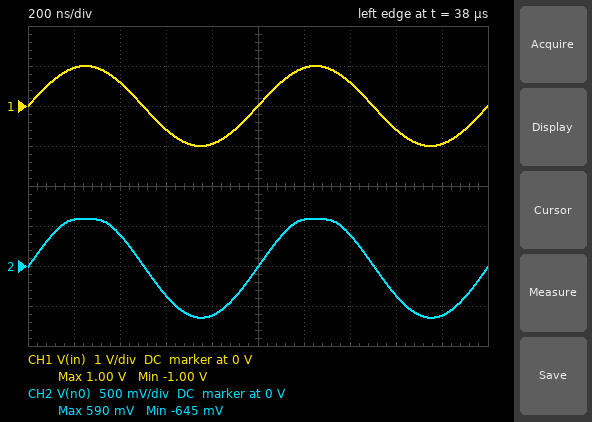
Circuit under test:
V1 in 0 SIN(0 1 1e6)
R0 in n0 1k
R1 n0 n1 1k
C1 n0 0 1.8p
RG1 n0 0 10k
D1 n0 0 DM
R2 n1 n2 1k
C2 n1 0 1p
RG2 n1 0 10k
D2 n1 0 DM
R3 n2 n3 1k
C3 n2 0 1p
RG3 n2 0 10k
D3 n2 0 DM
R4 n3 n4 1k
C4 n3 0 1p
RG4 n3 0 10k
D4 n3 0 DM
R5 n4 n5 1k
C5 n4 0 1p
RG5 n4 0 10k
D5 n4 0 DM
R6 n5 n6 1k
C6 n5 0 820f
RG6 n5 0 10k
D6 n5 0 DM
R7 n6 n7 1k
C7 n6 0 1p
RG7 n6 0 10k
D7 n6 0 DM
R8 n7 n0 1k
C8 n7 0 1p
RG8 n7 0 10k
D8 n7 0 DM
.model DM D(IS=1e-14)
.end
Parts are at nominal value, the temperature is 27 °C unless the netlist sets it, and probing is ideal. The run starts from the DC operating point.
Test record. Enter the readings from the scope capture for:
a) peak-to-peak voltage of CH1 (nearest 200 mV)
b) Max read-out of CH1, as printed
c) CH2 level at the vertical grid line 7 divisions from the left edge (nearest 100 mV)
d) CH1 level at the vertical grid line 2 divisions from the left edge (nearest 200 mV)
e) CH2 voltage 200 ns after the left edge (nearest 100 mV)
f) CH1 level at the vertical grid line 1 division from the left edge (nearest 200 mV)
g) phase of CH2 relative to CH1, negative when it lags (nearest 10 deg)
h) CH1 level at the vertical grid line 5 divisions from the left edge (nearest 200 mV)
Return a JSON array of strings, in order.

["2.0 V", "1.00 V", "400 mV", "600 mV", "600 mV", "1.0 V", "0 deg", "0 V"]
